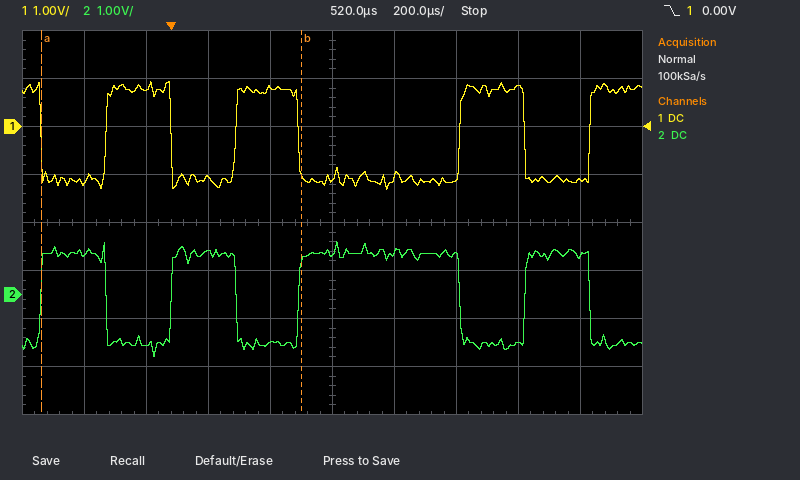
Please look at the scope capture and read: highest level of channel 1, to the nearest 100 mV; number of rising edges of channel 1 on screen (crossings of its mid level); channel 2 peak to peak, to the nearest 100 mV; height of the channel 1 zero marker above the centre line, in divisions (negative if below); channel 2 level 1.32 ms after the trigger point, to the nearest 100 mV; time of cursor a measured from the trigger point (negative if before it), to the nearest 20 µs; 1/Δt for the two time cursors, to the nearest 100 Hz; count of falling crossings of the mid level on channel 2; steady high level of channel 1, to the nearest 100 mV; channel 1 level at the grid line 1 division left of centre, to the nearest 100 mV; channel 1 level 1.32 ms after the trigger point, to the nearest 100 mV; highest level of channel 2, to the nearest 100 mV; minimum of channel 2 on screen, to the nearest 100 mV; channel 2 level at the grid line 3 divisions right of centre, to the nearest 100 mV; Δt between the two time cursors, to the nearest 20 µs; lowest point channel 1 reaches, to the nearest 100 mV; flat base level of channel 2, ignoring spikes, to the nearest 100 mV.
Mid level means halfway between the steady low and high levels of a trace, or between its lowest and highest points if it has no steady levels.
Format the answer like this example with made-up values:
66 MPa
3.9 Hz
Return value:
900 mV
4
2.4 V
+2.0 div
800 mV
-420 µs
1.2 kHz
4
800 mV
800 mV
-1.1 V
1.1 V
-1.3 V
-1.0 V
840 µs
-1.3 V
-1.0 V
